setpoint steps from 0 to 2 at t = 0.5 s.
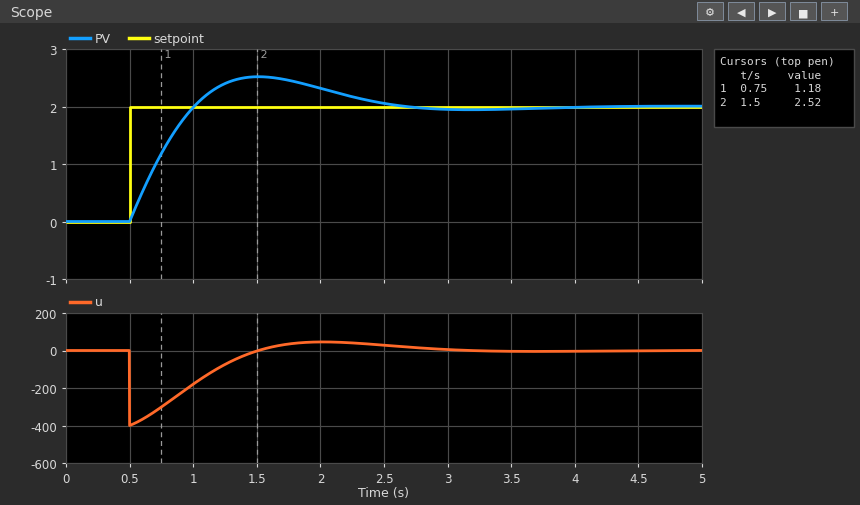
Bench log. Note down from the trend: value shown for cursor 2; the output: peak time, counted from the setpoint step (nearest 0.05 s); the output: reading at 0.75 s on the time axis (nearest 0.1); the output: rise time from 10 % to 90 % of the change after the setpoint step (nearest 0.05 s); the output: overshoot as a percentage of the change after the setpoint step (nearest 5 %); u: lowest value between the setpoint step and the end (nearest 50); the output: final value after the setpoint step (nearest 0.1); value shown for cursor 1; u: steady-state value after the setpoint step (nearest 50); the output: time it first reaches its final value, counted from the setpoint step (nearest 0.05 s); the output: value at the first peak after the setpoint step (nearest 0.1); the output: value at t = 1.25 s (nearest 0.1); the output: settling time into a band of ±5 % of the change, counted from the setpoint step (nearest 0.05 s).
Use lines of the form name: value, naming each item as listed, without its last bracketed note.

value shown for cursor 2: 2.52
the output: peak time, counted from the setpoint step: 1.00 s
the output: reading at 0.75 s on the time axis: 1.2
the output: rise time from 10 % to 90 % of the change after the setpoint step: 0.40 s
the output: overshoot as a percentage of the change after the setpoint step: 25 %
u: lowest value between the setpoint step and the end: -400
the output: final value after the setpoint step: 2.0
value shown for cursor 1: 1.18
u: steady-state value after the setpoint step: 0
the output: time it first reaches its final value, counted from the setpoint step: 0.50 s
the output: value at the first peak after the setpoint step: 2.5
the output: value at t = 1.25 s: 2.4
the output: settling time into a band of ±5 % of the change, counted from the setpoint step: 1.90 s
